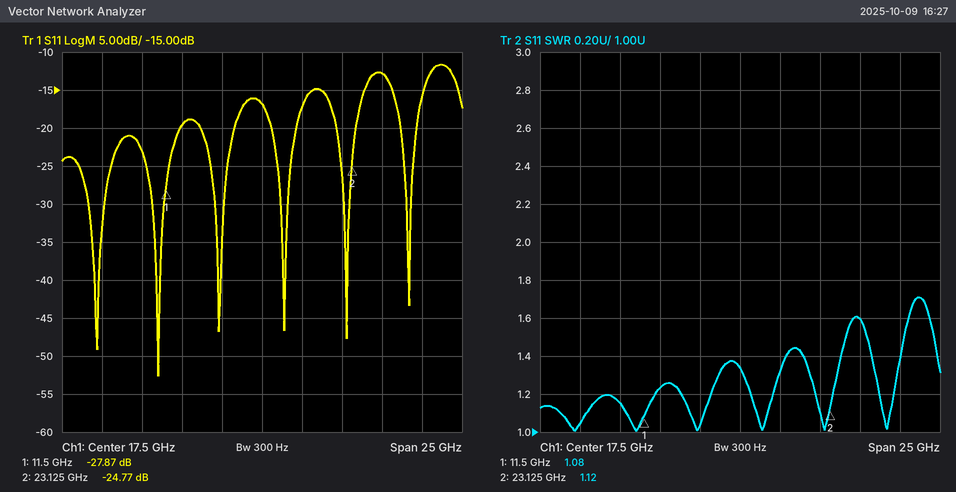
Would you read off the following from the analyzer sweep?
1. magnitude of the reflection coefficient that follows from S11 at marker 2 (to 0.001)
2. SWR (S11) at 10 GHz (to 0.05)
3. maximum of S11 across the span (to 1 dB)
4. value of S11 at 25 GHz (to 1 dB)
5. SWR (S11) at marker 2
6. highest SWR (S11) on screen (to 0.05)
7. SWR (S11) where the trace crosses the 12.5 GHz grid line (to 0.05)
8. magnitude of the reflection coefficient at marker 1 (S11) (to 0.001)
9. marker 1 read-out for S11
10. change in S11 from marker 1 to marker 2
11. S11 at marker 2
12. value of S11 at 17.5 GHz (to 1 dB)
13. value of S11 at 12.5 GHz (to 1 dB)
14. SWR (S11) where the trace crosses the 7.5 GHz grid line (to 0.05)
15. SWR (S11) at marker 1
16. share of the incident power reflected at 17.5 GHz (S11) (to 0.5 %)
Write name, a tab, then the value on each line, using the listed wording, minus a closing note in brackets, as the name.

magnitude of the reflection coefficient that follows from S11 at marker 2	0.058
SWR (S11) at 10 GHz	1.15
maximum of S11 across the span	-12 dB
value of S11 at 25 GHz	-13 dB
SWR (S11) at marker 2	1.12
highest SWR (S11) on screen	1.70
SWR (S11) where the trace crosses the 12.5 GHz grid line	1.25
magnitude of the reflection coefficient at marker 1 (S11)	0.040
marker 1 read-out for S11	-27.87 dB
change in S11 from marker 1 to marker 2	3.10 dB
S11 at marker 2	-24.77 dB
value of S11 at 17.5 GHz	-17 dB
value of S11 at 12.5 GHz	-20 dB
SWR (S11) where the trace crosses the 7.5 GHz grid line	1.05
SWR (S11) at marker 1	1.08
share of the incident power reflected at 17.5 GHz (S11)	2.0 %
